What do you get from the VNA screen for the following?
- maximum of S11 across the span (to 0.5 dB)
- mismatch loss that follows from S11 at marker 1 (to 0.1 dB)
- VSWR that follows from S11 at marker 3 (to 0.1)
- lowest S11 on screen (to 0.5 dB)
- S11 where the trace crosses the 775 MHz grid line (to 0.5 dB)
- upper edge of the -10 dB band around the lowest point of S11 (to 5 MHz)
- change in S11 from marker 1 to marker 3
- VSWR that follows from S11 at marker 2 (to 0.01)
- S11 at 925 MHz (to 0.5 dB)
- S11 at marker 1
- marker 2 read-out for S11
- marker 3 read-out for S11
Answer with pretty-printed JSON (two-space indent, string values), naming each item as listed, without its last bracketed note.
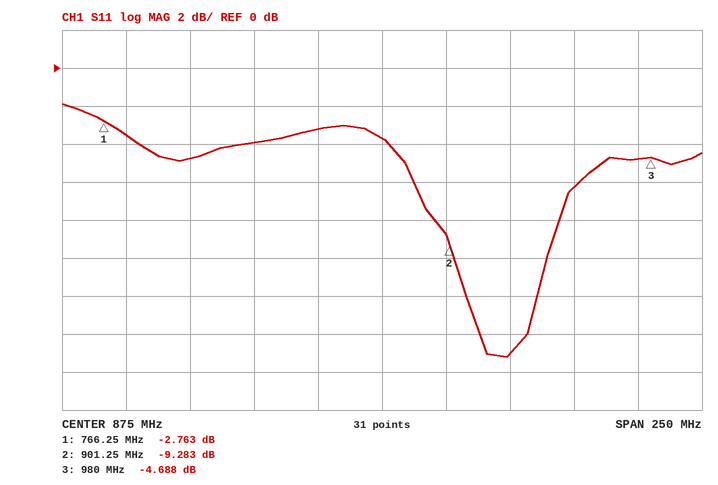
{
  "maximum of S11 across the span": "-2.0 dB",
  "mismatch loss that follows from S11 at marker 1": "3.3 dB",
  "VSWR that follows from S11 at marker 3": "3.8",
  "lowest S11 on screen": "-15.0 dB",
  "S11 where the trace crosses the 775 MHz grid line": "-3.5 dB",
  "upper edge of the -10 dB band around the lowest point of S11": "940 MHz",
  "change in S11 from marker 1 to marker 3": "-1.925 dB",
  "VSWR that follows from S11 at marker 2": "2.05",
  "S11 at 925 MHz": "-15.0 dB",
  "S11 at marker 1": "-2.763 dB",
  "marker 2 read-out for S11": "-9.283 dB",
  "marker 3 read-out for S11": "-4.688 dB"
}
